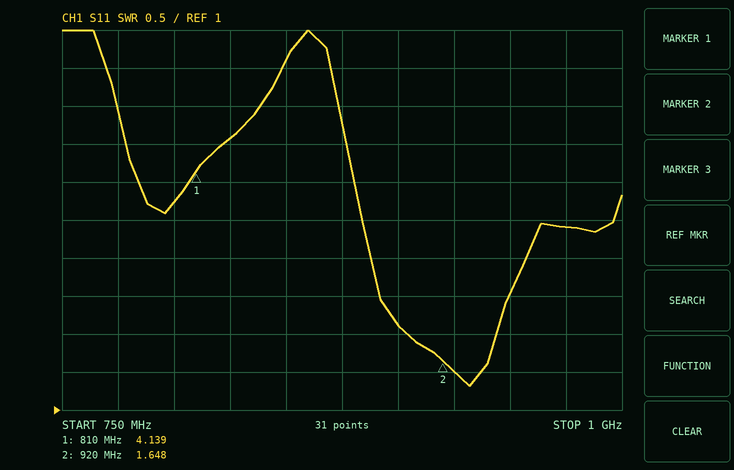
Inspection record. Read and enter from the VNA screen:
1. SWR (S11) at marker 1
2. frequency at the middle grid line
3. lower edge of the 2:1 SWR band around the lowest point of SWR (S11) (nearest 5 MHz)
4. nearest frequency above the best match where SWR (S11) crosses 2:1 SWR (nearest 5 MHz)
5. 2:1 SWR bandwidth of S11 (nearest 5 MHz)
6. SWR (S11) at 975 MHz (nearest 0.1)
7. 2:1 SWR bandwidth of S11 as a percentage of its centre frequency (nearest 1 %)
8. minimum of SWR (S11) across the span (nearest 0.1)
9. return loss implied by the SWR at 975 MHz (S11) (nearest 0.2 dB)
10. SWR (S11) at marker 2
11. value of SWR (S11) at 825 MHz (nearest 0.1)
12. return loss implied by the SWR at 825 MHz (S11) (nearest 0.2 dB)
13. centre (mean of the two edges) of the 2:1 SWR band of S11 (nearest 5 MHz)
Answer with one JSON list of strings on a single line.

["4.139", "875 MHz", "905 MHz", "945 MHz", "40 MHz", "3.4", "4 %", "1.3", "5.2 dB", "1.648", "4.6", "3.8 dB", "925 MHz"]
